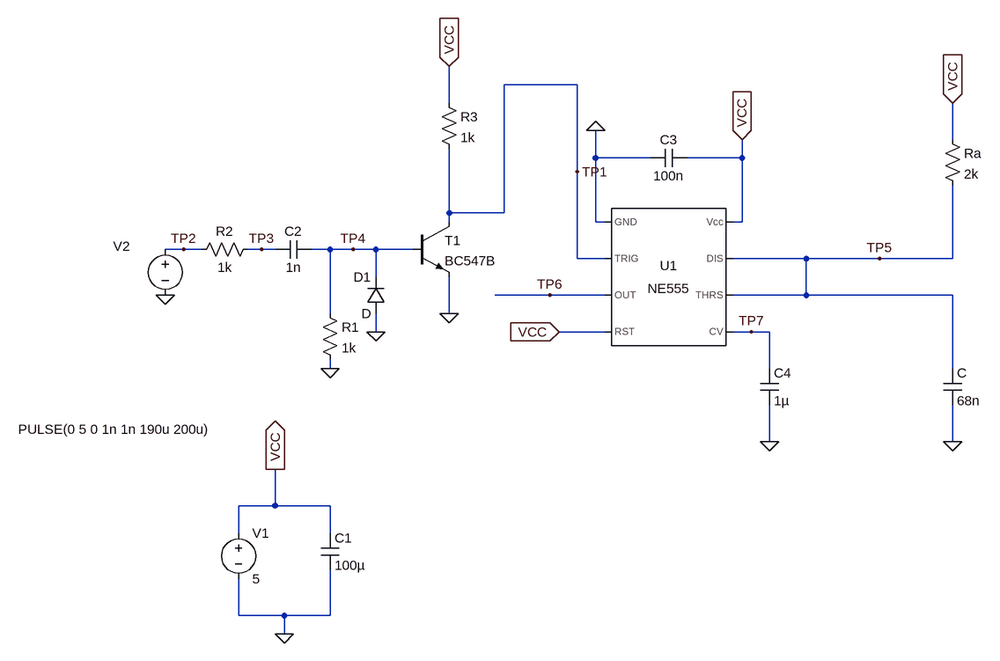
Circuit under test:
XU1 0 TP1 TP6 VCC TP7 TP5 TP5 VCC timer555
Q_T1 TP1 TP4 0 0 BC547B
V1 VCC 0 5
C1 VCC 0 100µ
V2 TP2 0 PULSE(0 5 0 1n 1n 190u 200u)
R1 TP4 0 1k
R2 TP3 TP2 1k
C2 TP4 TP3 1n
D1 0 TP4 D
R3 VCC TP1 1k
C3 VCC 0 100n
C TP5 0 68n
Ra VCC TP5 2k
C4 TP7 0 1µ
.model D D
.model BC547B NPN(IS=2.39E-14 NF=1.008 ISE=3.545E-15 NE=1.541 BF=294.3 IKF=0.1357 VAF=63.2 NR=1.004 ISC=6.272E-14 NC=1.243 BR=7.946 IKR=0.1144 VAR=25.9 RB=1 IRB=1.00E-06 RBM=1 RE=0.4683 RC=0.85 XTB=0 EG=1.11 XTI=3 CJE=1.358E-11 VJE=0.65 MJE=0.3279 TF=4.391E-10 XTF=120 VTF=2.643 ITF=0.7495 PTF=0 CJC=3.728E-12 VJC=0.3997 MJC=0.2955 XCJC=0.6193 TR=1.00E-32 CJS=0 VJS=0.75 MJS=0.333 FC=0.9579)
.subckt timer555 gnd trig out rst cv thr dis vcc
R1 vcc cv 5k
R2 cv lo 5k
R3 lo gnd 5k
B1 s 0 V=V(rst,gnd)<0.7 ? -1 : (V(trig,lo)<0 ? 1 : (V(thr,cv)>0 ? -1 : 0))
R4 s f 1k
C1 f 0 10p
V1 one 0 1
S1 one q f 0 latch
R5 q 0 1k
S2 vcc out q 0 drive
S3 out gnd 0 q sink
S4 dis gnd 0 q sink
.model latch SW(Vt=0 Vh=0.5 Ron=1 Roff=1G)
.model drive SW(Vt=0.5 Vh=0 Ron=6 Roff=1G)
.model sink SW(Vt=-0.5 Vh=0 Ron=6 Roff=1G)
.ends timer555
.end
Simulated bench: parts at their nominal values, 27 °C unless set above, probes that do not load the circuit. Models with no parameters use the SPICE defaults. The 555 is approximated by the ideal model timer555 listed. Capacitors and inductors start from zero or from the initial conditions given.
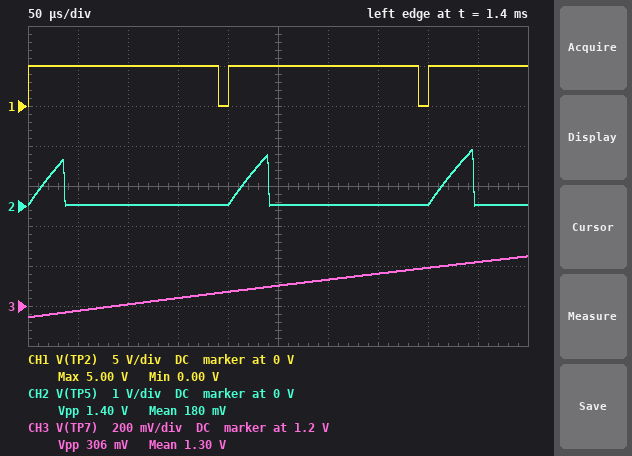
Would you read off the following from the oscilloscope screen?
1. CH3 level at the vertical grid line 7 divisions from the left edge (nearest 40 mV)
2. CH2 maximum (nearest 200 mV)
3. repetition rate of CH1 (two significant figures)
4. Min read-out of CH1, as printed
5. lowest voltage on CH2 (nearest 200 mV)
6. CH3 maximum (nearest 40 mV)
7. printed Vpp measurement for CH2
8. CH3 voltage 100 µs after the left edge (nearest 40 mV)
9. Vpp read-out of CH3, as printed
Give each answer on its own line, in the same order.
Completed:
1.36 V
1.4 V
5.0 kHz
0.00 V
0 V
1.44 V
1.40 V
1.20 V
306 mV
